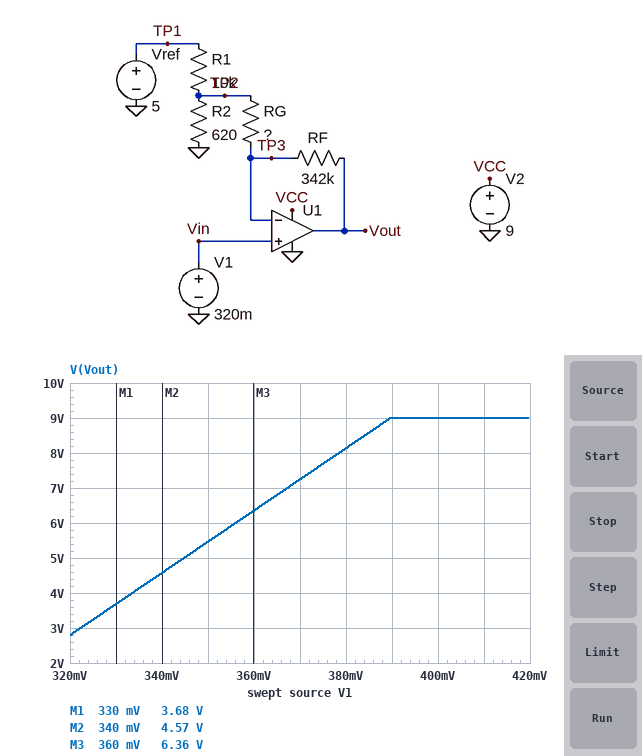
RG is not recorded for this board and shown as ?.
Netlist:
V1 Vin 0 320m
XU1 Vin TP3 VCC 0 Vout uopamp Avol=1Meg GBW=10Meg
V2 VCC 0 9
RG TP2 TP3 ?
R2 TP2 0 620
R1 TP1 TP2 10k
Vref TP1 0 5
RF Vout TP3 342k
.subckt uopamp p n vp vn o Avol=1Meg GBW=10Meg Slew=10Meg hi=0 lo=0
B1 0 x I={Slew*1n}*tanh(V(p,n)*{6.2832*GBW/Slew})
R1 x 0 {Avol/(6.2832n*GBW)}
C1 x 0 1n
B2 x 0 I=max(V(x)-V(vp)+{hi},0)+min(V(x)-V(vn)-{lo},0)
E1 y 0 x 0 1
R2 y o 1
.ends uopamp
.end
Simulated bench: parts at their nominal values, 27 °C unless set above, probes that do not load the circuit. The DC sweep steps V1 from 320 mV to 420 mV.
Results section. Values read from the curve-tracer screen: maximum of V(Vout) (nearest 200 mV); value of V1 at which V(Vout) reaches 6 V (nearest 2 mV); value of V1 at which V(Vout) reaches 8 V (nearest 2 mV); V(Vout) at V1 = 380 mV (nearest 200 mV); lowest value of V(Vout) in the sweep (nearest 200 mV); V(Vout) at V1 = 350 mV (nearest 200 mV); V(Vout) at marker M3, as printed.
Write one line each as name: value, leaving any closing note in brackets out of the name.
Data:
maximum of V(Vout): 9.0 V
value of V1 at which V(Vout) reaches 6 V: 356 mV
value of V1 at which V(Vout) reaches 8 V: 378 mV
V(Vout) at V1 = 380 mV: 8.2 V
lowest value of V(Vout) in the sweep: 2.8 V
V(Vout) at V1 = 350 mV: 5.4 V
V(Vout) at marker M3, as printed: 6.36 V
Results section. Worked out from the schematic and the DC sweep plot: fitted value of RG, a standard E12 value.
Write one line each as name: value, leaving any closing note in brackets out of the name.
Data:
fitted value of RG, a standard E12 value: 3.3 kΩ
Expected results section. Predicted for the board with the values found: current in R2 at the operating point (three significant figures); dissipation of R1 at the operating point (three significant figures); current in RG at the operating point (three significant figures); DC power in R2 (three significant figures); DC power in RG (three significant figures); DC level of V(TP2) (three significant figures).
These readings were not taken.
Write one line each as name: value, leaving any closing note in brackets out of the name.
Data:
current in R2 at the operating point: 478 µA
dissipation of R1 at the operating point: 2.21 mW
current in RG at the operating point: 7.23 µA
DC power in R2: 141 µW
DC power in RG: 173 nW
DC level of V(TP2): 296 mV
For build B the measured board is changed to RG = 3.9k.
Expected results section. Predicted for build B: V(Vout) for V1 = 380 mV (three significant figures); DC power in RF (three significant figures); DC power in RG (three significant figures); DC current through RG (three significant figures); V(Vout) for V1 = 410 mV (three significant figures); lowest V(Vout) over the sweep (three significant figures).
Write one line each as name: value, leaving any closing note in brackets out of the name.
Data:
V(Vout) for V1 = 380 mV: 7.10 V
DC power in RF: 13.4 µW
DC power in RG: 153 nW
DC current through RG: 6.27 µA
V(Vout) for V1 = 410 mV: 9.00 V
lowest V(Vout) over the sweep: 2.46 V
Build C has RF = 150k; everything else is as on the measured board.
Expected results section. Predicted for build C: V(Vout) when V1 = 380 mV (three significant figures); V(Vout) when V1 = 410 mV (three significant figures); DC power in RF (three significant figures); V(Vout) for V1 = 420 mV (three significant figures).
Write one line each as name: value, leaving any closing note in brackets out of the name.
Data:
V(Vout) when V1 = 380 mV: 3.78 V
V(Vout) when V1 = 410 mV: 4.97 V
DC power in RF: 7.85 µW
V(Vout) for V1 = 420 mV: 5.37 V
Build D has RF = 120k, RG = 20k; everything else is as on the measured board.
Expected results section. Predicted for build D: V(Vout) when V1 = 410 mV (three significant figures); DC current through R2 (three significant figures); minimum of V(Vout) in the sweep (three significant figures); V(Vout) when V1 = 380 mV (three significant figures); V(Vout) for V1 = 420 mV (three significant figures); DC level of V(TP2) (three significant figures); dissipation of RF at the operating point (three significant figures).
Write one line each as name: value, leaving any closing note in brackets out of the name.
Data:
V(Vout) when V1 = 410 mV: 1.10 V
DC current through R2: 472 µA
minimum of V(Vout) in the sweep: 484 mV
V(Vout) when V1 = 380 mV: 894 mV
V(Vout) for V1 = 420 mV: 1.17 V
DC level of V(TP2): 293 mV
dissipation of RF at the operating point: 224 nW
